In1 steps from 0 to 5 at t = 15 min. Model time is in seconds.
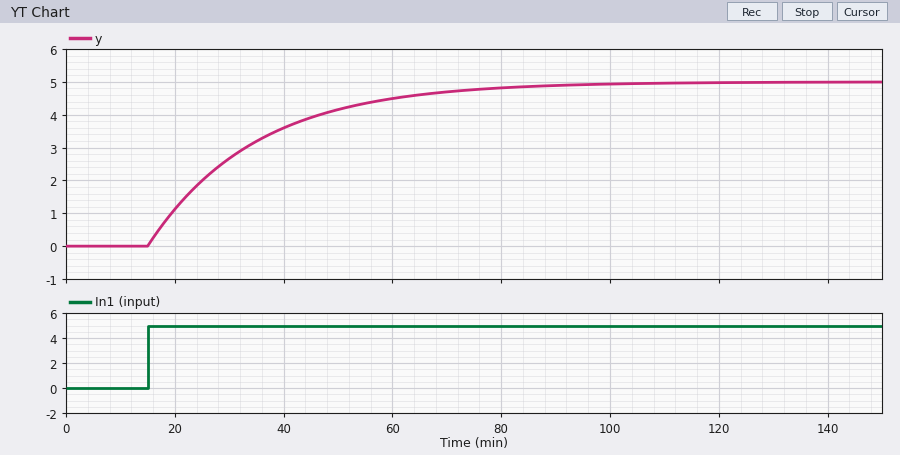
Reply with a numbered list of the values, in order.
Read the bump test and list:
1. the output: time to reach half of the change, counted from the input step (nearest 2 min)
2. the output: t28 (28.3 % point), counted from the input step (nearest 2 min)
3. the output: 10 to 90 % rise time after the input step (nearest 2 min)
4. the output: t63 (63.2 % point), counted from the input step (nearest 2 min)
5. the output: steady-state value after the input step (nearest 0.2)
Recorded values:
1. 14 min
2. 6 min
3. 44 min
4. 20 min
5. 5.0
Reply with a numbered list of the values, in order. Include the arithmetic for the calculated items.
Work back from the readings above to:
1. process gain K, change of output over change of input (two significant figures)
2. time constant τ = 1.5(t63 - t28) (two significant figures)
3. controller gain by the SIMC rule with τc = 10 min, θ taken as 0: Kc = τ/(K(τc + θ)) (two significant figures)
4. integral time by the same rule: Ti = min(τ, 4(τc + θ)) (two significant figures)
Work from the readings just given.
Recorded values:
1. (5 - 0) / 5 = 1.0
2. 1.5 × (20 - 6) = 21 min
3. 21 / (1 × (10 + 0)) = 2.1
4. min(21, 4 × (10 + 0)) = 21 min
